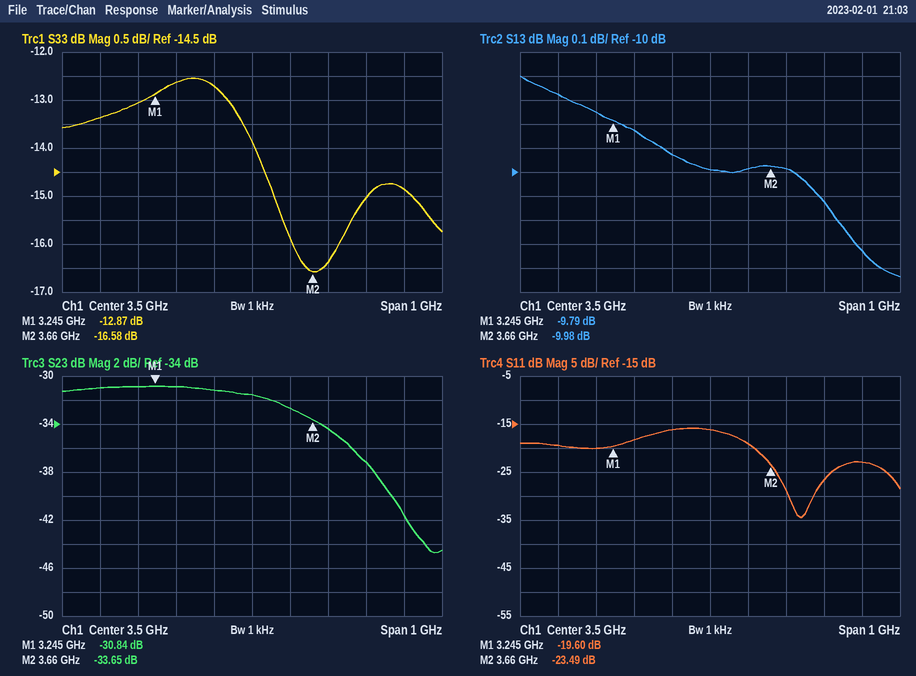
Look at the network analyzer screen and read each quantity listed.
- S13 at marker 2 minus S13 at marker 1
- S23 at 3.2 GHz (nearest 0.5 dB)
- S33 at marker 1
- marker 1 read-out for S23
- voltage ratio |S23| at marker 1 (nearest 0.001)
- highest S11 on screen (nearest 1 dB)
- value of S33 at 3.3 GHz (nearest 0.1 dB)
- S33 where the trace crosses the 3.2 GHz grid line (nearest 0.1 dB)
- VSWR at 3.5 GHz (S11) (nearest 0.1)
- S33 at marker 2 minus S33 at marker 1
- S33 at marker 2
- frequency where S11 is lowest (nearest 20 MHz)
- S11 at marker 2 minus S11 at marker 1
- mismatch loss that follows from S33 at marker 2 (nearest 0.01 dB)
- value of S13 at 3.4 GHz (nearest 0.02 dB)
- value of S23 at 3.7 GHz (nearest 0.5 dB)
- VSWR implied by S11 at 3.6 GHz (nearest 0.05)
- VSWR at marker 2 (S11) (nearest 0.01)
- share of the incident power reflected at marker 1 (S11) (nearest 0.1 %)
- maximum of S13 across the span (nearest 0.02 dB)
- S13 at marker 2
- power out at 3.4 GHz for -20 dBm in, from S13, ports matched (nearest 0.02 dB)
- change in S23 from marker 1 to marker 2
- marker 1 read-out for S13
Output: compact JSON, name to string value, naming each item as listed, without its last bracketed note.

{"S13 at marker 2 minus S13 at marker 1": "-0.19 dB", "S23 at 3.2 GHz": "-31.0 dB", "S33 at marker 1": "-12.87 dB", "marker 1 read-out for S23": "-30.84 dB", "voltage ratio |S23| at marker 1": "0.029", "highest S11 on screen": "-16 dB", "value of S33 at 3.3 GHz": "-12.6 dB", "S33 where the trace crosses the 3.2 GHz grid line": "-13.1 dB", "VSWR at 3.5 GHz (S11)": "1.4", "S33 at marker 2 minus S33 at marker 1": "-3.71 dB", "S33 at marker 2": "-16.58 dB", "frequency where S11 is lowest": "3.74 GHz", "S11 at marker 2 minus S11 at marker 1": "-3.89 dB", "mismatch loss that follows from S33 at marker 2": "0.10 dB", "value of S13 at 3.4 GHz": "-9.92 dB", "value of S23 at 3.7 GHz": "-34.5 dB", "VSWR implied by S11 at 3.6 GHz": "1.25", "VSWR at marker 2 (S11)": "1.14", "share of the incident power reflected at marker 1 (S11)": "1.1 %", "maximum of S13 across the span": "-9.60 dB", "S13 at marker 2": "-9.98 dB", "power out at 3.4 GHz for -20 dBm in, from S13, ports matched": "-29.92 dBm", "change in S23 from marker 1 to marker 2": "-2.81 dB", "marker 1 read-out for S13": "-9.79 dB"}
